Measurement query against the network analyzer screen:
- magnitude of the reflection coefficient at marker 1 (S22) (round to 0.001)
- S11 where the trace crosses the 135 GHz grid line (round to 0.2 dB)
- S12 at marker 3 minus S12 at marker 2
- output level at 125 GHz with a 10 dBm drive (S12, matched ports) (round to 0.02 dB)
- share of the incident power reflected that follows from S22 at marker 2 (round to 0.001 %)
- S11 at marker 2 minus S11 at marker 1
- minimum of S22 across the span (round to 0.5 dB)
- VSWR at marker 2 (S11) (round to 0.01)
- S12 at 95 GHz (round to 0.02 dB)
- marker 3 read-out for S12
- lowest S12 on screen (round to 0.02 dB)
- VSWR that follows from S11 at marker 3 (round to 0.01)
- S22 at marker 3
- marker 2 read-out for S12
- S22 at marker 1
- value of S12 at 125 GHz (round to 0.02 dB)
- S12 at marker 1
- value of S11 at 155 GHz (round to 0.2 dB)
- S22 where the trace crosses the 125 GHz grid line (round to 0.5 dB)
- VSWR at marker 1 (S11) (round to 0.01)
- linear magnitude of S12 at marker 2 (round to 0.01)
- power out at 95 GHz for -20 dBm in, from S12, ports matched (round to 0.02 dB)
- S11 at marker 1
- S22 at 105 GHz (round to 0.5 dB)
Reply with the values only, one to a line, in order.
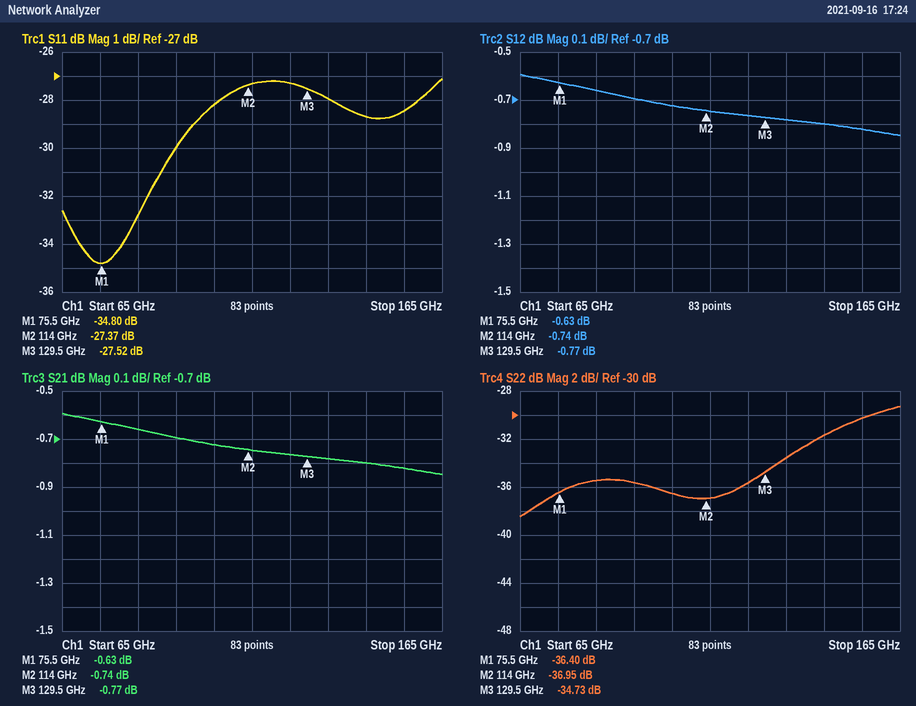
0.015
-28.0 dB
-0.03 dB
9.24 dBm
0.020 %
7.43 dB
-38.5 dB
1.09
-0.70 dB
-0.77 dB
-0.84 dB
1.09
-34.73 dB
-0.74 dB
-36.40 dB
-0.76 dB
-0.63 dB
-28.4 dB
-35.5 dB
1.04
0.92
-20.70 dBm
-34.80 dB
-36.5 dB
